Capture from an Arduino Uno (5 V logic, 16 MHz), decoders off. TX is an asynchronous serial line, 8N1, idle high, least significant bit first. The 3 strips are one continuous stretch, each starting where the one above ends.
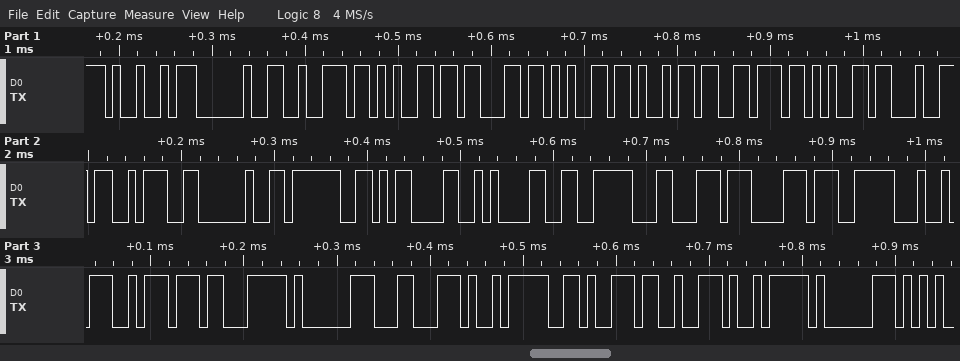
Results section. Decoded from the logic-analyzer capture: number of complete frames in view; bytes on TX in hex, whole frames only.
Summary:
29
0x49 0x20 0x72 0x65 0x63 0x65 0x69 0x76 0x65 0x64 0x3A 0x20 0x3F 0x0D 0x0A 0xE6 0x8C 0x87 0xE7 0xA4 0xBA 0xE3 0x81 0x8C 0xE9 0x96 0x93 0xE9 0x81
